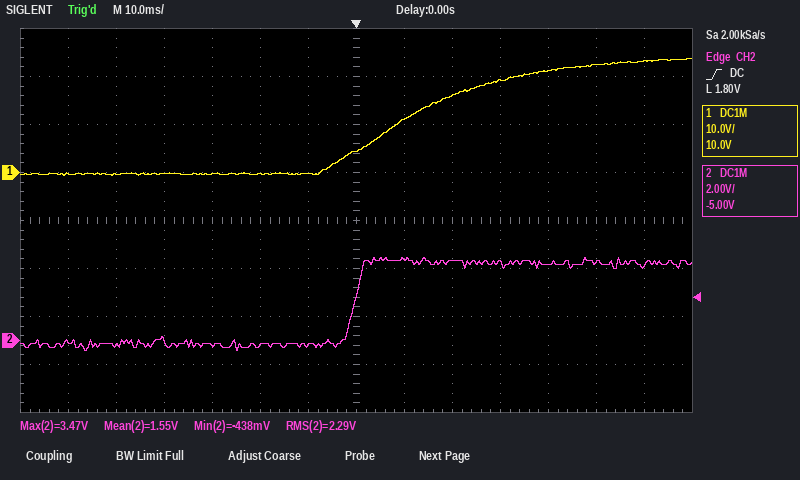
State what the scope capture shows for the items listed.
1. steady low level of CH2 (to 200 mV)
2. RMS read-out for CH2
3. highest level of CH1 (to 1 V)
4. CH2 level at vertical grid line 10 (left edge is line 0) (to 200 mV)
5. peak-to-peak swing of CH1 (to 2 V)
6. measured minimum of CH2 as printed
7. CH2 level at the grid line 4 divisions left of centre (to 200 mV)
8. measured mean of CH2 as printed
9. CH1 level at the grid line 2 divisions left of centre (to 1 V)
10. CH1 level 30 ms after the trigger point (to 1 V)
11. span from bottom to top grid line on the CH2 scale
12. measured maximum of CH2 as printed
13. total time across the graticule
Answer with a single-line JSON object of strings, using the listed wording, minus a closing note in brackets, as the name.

{"steady low level of CH2": "-200 mV", "RMS read-out for CH2": "2.29 V", "highest level of CH1": "24 V", "CH2 level at vertical grid line 10 (left edge is line 0)": "3.2 V", "peak-to-peak swing of CH1": "24 V", "measured minimum of CH2 as printed": "-438 mV", "CH2 level at the grid line 4 divisions left of centre": "0.0 V", "measured mean of CH2 as printed": "1.55 V", "CH1 level at the grid line 2 divisions left of centre": "0 V", "CH1 level 30 ms after the trigger point": "19 V", "span from bottom to top grid line on the CH2 scale": "16 V", "measured maximum of CH2 as printed": "3.47 V", "total time across the graticule": "140 ms"}
